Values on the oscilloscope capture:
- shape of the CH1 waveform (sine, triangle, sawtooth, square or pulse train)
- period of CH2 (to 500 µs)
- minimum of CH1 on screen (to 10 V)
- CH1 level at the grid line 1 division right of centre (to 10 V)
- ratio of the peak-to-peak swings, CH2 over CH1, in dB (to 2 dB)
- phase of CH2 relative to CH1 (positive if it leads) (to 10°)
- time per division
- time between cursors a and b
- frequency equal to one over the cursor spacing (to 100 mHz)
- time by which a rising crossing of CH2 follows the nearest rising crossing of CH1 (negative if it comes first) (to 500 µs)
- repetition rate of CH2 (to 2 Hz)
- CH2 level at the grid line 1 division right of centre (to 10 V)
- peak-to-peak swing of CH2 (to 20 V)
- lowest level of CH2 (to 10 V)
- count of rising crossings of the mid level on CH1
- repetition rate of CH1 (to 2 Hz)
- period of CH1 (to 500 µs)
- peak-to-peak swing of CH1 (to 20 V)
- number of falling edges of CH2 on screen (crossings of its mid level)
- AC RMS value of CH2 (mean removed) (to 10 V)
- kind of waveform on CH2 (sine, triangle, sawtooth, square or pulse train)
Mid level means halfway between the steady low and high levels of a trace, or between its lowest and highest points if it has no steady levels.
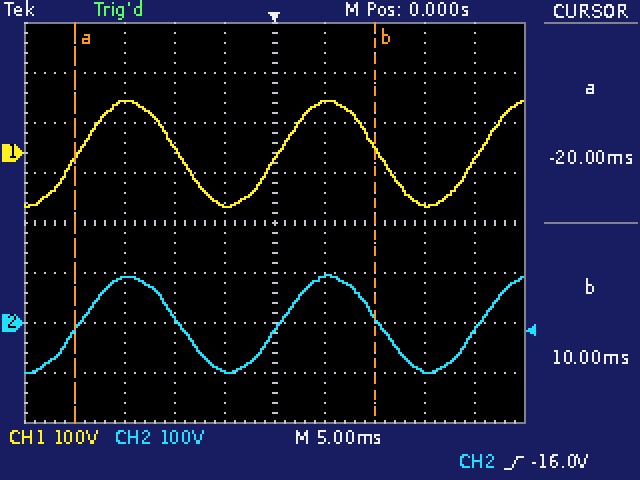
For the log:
sine
20.0 ms
-110 V
100 V
0 dB
0°
5 ms
30.0 ms
33.3 Hz
0.0 ms
50 Hz
90 V
200 V
-100 V
3
50 Hz
20.0 ms
220 V
2
70 V
sine
